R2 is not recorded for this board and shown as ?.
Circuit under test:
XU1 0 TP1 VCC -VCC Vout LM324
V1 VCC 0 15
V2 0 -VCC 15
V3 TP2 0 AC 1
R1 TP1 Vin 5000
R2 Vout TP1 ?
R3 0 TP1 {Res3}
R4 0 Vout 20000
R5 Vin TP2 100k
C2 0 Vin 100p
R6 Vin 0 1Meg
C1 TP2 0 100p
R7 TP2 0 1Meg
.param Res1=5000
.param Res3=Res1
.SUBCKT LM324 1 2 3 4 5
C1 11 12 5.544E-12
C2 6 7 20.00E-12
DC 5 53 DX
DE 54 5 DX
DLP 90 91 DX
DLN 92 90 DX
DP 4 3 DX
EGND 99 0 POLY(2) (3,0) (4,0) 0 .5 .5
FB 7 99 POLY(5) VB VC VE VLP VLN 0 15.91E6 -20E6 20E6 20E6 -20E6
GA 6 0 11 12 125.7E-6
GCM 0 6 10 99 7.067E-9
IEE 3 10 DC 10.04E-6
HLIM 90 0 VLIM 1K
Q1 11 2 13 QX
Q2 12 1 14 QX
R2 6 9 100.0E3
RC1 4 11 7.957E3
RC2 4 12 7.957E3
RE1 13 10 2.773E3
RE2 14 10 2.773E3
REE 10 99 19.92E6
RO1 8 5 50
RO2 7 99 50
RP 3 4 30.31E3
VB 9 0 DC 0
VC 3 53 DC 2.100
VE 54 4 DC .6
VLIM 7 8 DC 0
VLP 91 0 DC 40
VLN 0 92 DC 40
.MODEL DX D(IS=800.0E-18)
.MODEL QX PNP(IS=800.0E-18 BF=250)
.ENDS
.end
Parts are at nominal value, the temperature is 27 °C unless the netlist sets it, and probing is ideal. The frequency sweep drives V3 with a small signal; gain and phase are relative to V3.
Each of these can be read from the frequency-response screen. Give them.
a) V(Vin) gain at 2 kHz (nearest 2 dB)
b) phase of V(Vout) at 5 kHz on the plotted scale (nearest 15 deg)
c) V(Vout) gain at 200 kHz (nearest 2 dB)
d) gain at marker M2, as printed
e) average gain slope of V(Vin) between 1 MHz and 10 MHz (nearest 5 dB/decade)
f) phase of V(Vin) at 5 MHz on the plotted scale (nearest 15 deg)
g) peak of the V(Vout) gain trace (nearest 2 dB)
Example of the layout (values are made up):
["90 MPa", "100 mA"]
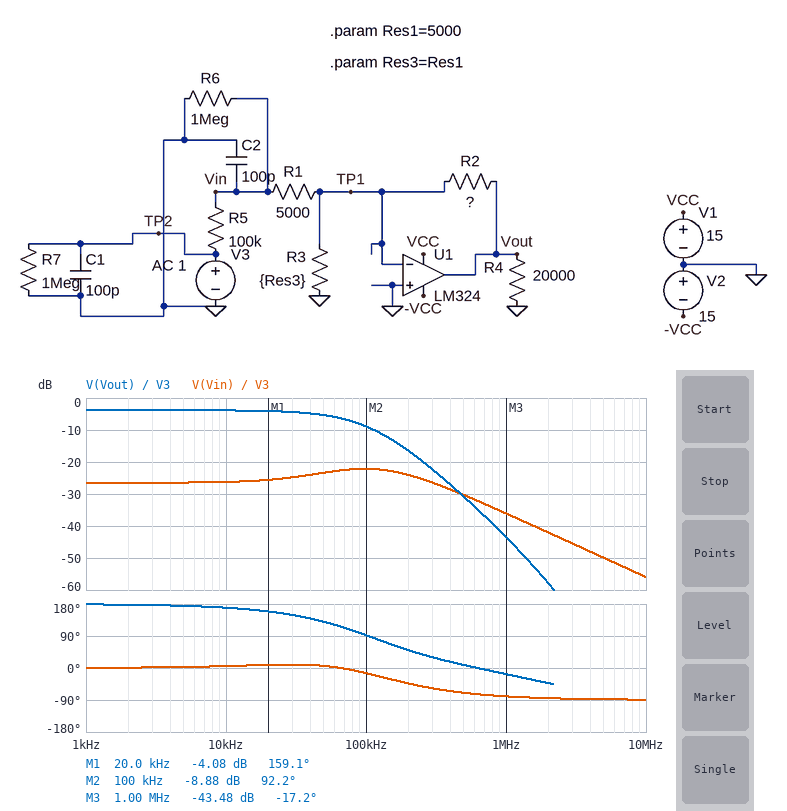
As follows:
["-26 dB", "180 deg", "-16 dB", "-8.88 dB", "-20 dB/decade", "-90 deg", "-4 dB"]
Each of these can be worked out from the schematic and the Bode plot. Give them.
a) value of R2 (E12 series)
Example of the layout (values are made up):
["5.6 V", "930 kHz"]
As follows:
["68 kΩ"]
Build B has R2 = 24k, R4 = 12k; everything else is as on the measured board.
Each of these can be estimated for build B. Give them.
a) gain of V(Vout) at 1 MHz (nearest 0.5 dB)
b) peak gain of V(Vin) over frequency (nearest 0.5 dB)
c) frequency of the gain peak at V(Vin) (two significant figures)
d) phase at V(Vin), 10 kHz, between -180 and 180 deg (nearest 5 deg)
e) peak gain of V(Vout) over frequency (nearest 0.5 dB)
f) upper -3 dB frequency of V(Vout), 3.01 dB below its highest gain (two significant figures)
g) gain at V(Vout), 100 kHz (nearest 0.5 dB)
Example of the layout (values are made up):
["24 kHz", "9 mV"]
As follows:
["-44.0 dB", "-23.5 dB", "150 kHz", "0 deg", "-13.0 dB", "160 kHz", "-13.5 dB"]
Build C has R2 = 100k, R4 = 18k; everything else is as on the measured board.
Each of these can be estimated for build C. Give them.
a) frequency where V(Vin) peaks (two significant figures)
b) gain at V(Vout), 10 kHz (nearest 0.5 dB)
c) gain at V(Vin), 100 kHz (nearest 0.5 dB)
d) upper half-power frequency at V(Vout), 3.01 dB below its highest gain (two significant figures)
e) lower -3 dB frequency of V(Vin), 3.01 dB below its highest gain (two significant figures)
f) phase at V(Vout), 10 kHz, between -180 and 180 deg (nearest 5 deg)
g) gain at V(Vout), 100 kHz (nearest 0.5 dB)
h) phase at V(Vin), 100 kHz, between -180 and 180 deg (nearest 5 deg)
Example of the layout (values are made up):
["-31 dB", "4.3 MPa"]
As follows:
["82 kHz", "-0.5 dB", "-22.0 dB", "50 kHz", "21 kHz", "165 deg", "-8.5 dB", "-20 deg"]
